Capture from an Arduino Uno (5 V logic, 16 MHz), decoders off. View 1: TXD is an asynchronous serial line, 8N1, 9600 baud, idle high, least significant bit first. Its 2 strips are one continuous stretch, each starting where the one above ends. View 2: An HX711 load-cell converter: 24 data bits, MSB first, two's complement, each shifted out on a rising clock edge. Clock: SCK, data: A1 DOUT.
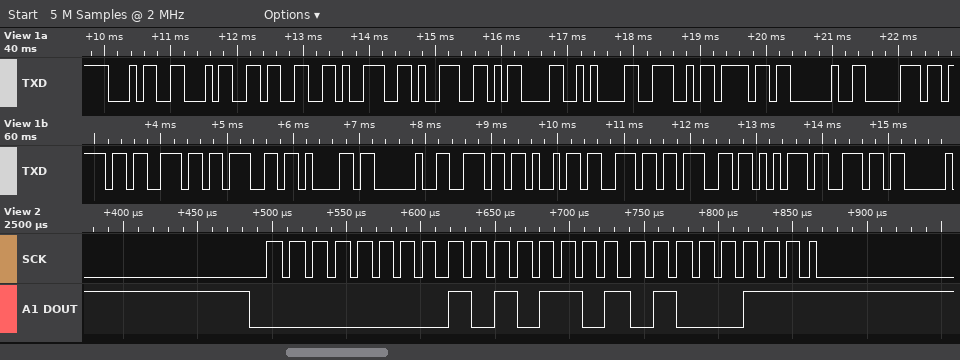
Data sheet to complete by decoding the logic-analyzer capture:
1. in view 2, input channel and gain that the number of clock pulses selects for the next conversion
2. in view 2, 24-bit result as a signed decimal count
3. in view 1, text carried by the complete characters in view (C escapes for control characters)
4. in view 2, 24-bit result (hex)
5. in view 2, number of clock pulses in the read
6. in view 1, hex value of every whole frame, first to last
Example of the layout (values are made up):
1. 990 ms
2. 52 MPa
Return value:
1. channel A, gain 128
2. 44359
3. "44399\r\nNo ponga ningun"
4. 0x00AD47
5. 25
6. 0x34 0x34 0x33 0x39 0x39 0x0D 0x0A 0x4E 0x6F 0x20 0x70 0x6F 0x6E 0x67 0x61 0x20 0x6E 0x69 0x6E 0x67 0x75 0x6E
